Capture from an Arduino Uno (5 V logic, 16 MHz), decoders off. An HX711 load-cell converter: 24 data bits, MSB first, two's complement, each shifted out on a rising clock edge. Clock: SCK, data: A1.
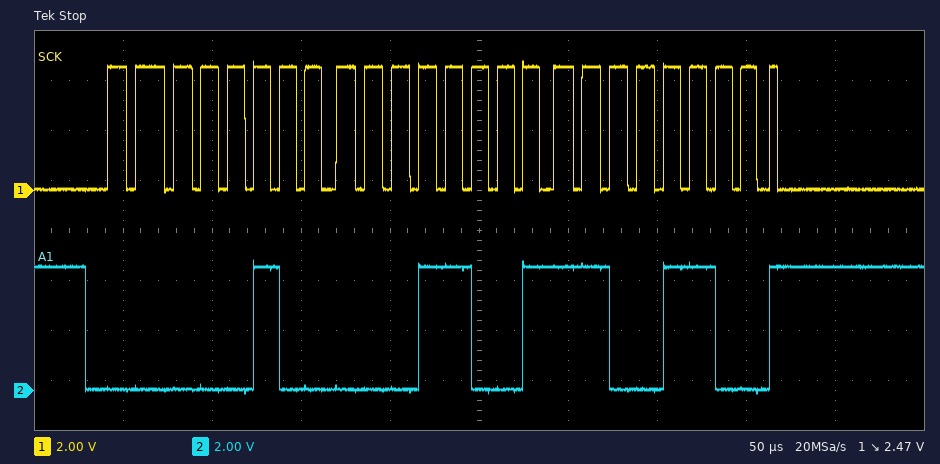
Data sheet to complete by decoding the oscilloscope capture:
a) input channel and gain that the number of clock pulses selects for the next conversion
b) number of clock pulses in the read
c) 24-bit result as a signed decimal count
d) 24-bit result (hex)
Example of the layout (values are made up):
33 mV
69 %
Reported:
channel A, gain 128
25
268748
0x0419CC
